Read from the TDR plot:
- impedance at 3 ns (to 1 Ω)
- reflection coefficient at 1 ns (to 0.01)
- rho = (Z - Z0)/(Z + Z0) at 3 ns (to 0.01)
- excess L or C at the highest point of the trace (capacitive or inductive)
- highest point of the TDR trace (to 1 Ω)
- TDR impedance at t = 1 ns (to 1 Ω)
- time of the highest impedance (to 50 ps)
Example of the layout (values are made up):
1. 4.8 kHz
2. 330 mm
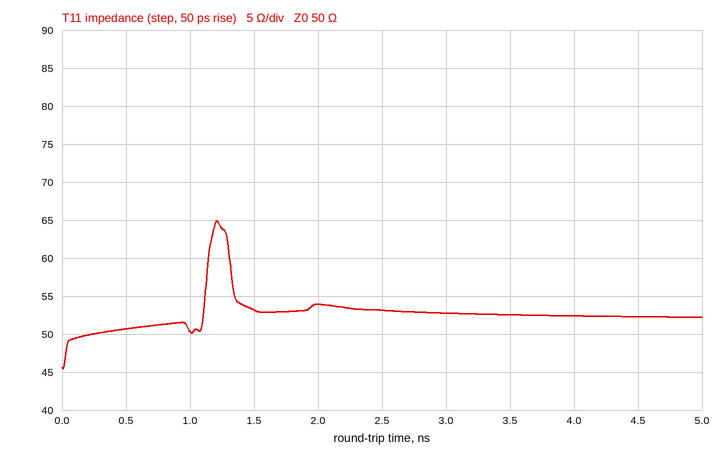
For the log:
1. 53 Ω
2. 0.00
3. +0.03
4. inductive
5. 65 Ω
6. 50 Ω
7. 1.20 ns
